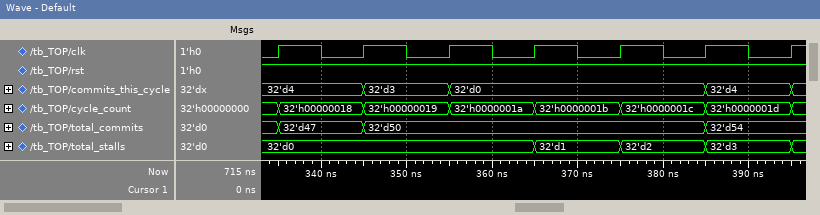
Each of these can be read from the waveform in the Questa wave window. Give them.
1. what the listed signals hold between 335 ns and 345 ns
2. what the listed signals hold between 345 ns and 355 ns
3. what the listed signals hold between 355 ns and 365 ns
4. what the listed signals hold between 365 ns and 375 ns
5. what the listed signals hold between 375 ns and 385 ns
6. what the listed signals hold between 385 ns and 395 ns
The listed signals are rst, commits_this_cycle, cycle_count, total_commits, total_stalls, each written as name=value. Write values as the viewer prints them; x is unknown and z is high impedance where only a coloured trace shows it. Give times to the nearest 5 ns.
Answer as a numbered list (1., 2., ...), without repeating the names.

1. rst=1, commits_this_cycle=32'd4, cycle_count=32'h00000018, total_commits=32'd47, total_stalls=32'd0
2. rst=1, commits_this_cycle=32'd3, cycle_count=32'h00000019, total_commits=32'd50, total_stalls=32'd0
3. rst=1, commits_this_cycle=32'd0, cycle_count=32'h0000001a, total_commits=32'd50, total_stalls=32'd0
4. rst=1, commits_this_cycle=32'd0, cycle_count=32'h0000001b, total_commits=32'd50, total_stalls=32'd1
5. rst=1, commits_this_cycle=32'd0, cycle_count=32'h0000001c, total_commits=32'd50, total_stalls=32'd2
6. rst=1, commits_this_cycle=32'd4, cycle_count=32'h0000001d, total_commits=32'd54, total_stalls=32'd3
